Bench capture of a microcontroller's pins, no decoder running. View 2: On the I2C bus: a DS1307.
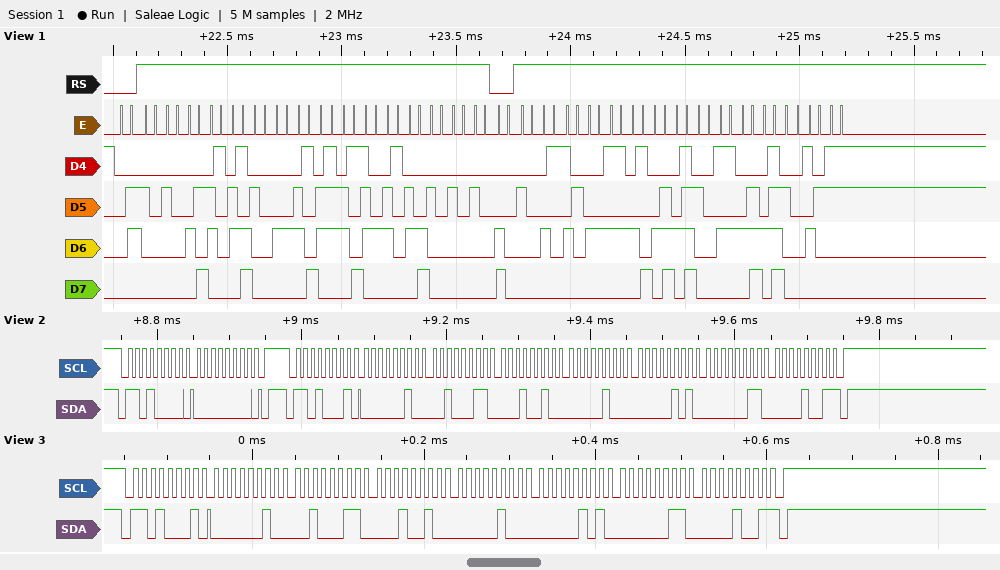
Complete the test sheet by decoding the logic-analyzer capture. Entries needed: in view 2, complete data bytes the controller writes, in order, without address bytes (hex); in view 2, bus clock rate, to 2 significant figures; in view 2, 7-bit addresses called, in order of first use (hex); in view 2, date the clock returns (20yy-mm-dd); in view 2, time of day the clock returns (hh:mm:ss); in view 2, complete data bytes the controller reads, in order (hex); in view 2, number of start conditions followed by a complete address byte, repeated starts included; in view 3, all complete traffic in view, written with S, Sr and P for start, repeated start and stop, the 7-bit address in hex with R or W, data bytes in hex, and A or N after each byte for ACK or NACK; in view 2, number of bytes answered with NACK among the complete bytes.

00
100 kHz
0x68
2009-03-05
12:23:02
02 23 12 04 05 03 09
2
S 68R A 02 A 23 A 12 A 04 A 05 A 03 A 09 N P
1
